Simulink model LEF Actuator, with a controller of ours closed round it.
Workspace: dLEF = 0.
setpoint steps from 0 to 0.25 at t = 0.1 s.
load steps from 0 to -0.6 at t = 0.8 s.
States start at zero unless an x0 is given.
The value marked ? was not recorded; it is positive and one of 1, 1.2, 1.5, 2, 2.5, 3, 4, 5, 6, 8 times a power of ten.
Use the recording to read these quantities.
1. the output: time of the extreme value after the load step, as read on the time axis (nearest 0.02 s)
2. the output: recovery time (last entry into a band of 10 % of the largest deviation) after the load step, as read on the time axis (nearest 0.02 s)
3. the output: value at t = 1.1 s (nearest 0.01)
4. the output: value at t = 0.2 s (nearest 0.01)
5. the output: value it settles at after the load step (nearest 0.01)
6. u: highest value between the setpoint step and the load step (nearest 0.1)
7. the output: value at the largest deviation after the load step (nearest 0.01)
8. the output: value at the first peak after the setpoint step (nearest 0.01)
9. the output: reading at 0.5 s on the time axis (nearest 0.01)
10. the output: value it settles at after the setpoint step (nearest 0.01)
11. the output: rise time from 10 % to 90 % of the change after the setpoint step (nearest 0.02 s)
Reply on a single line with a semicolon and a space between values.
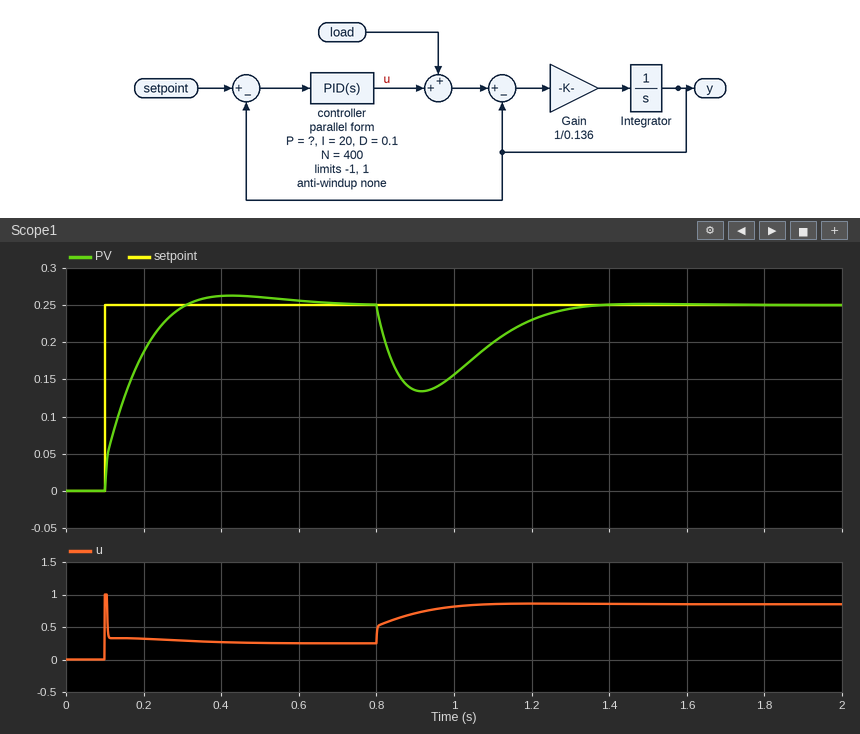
0.92 s; 1.24 s; 0.20; 0.19; 0.25; 1.0; 0.13; 0.26; 0.26; 0.25; 0.14 s
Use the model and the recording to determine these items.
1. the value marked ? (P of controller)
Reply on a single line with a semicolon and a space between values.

2.5
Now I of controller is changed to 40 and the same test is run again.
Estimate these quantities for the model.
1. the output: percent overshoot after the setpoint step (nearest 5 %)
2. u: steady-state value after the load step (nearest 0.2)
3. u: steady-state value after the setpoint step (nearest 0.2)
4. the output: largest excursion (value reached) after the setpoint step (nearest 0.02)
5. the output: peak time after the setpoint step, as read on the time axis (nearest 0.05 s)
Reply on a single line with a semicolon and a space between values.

15 %; 0.8; 0.2; 0.28; 0.30 s
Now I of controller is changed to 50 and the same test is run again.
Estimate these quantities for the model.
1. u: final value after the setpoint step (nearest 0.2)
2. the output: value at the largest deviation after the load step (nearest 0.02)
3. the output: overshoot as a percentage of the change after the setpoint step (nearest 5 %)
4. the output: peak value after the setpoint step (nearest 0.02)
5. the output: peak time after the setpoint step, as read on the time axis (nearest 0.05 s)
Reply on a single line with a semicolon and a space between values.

0.2; 0.16; 20 %; 0.30; 0.30 s
